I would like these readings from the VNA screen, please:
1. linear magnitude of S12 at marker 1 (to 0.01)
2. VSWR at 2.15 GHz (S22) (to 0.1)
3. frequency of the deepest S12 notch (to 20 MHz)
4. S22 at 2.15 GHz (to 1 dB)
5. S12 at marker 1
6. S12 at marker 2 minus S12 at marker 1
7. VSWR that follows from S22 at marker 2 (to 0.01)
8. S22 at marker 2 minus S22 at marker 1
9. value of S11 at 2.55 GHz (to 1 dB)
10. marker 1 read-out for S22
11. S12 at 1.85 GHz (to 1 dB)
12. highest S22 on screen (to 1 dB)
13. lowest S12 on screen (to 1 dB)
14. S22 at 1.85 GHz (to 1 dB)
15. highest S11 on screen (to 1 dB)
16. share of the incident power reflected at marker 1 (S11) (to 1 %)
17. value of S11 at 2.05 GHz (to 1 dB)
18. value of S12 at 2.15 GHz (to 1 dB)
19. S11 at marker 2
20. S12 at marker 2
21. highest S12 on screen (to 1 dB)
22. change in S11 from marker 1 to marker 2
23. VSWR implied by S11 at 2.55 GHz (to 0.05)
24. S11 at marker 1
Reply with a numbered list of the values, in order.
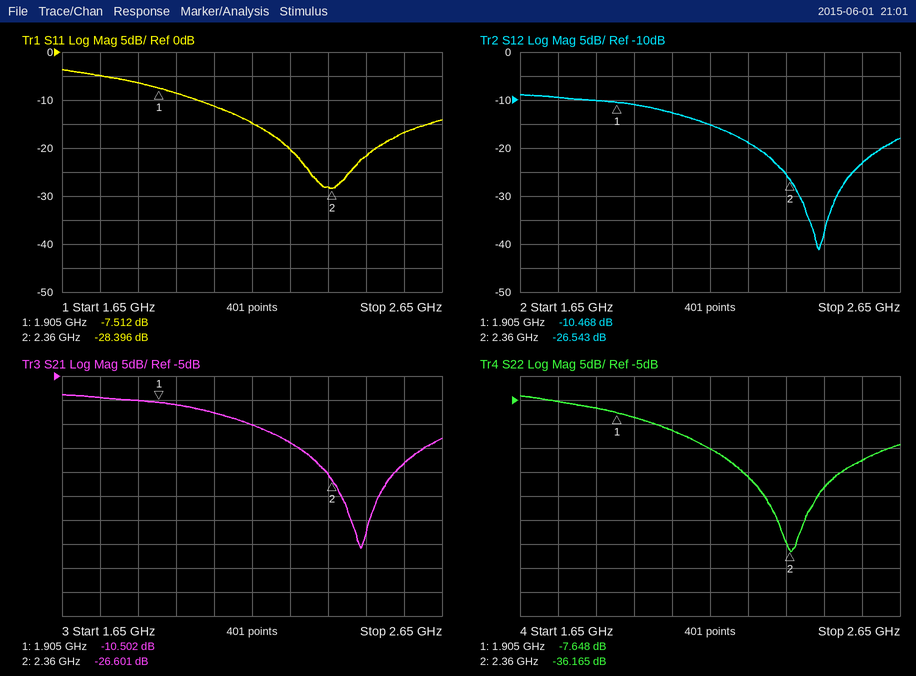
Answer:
1. 0.30
2. 1.4
3. 2.44 GHz
4. -15 dB
5. -10.468 dB
6. -16.075 dB
7. 1.03
8. -28.517 dB
9. -17 dB
10. -7.648 dB
11. -10 dB
12. -4 dB
13. -41 dB
14. -7 dB
15. -4 dB
16. 18 %
17. -11 dB
18. -15 dB
19. -28.396 dB
20. -26.543 dB
21. -9 dB
22. -20.884 dB
23. 1.35
24. -7.512 dB
